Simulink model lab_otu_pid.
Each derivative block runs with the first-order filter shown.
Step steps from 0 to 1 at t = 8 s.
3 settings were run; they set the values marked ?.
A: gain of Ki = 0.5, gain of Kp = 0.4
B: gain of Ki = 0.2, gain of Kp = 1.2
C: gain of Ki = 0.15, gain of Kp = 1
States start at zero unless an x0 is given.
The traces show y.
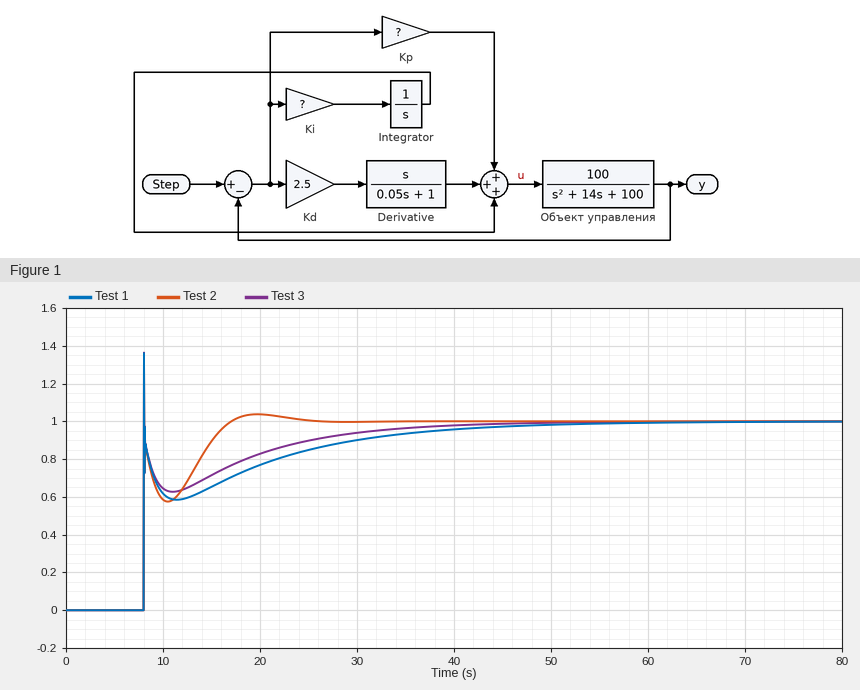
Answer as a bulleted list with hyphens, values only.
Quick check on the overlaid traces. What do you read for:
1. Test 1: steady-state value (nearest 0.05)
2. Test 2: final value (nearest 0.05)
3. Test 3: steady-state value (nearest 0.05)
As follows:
- 1.00
- 1.00
- 1.00
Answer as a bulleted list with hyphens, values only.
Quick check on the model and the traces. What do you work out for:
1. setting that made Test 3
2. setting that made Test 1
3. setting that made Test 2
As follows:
- B
- C
- A
